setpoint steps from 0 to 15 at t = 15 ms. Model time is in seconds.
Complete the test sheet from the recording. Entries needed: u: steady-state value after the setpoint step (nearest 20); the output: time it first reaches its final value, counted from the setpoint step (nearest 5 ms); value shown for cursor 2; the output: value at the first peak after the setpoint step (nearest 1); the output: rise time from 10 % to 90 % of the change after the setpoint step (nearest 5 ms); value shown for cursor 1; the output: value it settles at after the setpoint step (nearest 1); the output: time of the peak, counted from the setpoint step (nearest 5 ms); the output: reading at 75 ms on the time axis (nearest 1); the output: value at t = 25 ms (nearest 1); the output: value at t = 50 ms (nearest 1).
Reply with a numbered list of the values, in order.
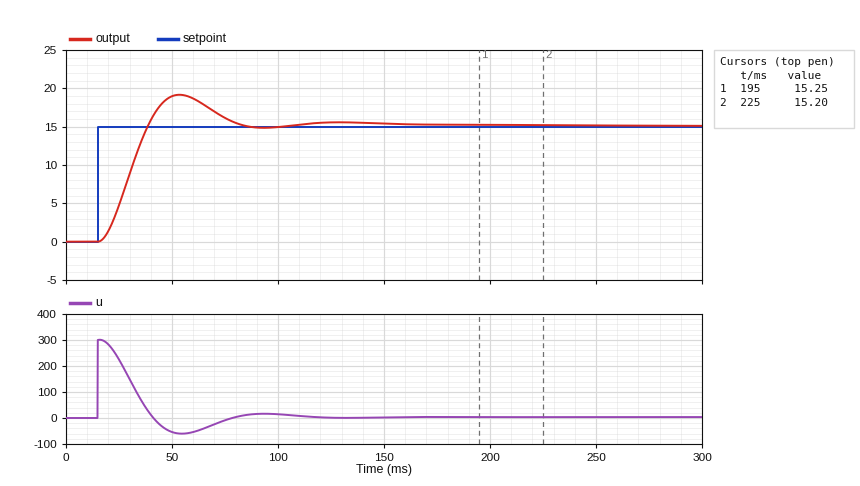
1. 0
2. 25 ms
3. 15.20
4. 19
5. 15 ms
6. 15.25
7. 15
8. 40 ms
9. 16
10. 5
11. 19
